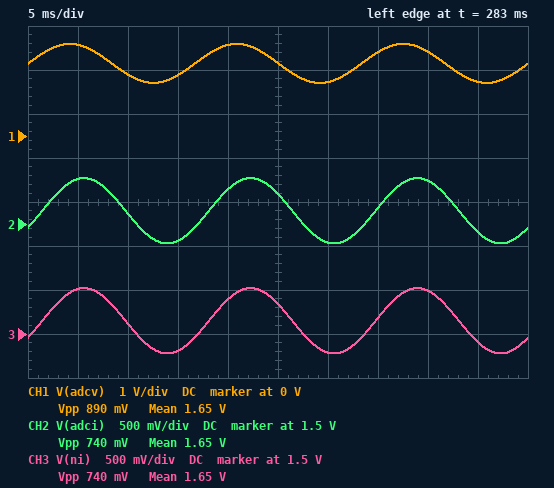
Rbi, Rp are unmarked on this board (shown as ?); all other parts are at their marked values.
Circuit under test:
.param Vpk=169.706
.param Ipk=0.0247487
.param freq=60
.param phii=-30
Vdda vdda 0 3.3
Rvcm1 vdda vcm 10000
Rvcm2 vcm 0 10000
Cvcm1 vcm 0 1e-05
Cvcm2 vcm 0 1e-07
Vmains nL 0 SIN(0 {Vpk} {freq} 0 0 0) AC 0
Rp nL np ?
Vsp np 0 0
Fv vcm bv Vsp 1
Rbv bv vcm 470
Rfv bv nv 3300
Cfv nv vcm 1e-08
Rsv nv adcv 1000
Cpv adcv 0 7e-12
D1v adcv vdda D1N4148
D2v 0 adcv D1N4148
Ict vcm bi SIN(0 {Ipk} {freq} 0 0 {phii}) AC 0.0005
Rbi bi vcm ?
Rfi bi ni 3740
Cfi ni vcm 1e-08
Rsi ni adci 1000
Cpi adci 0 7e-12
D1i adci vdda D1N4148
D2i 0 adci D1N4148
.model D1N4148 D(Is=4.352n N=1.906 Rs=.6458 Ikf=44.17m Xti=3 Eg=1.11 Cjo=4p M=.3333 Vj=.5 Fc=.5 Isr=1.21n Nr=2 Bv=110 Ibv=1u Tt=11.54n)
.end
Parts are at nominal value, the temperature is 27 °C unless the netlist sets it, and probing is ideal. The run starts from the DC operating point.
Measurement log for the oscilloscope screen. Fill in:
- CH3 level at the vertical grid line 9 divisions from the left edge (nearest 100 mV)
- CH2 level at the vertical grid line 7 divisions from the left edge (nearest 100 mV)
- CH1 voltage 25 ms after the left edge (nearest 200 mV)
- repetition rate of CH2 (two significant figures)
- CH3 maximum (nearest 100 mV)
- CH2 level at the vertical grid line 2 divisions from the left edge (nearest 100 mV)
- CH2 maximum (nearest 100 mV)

1.4 V
1.7 V
1.6 V
60 Hz
2.0 V
1.6 V
2.0 V
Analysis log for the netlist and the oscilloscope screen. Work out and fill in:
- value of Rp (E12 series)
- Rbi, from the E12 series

180 kΩ
15 Ω
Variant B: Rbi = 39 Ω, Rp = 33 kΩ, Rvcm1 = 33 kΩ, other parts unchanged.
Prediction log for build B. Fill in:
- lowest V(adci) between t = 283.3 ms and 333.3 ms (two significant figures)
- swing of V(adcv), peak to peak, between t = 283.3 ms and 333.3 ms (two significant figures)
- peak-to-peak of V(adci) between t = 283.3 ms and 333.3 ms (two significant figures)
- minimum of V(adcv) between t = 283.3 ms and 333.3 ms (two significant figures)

85 mV
4.0 V
1.9 V
-520 mV
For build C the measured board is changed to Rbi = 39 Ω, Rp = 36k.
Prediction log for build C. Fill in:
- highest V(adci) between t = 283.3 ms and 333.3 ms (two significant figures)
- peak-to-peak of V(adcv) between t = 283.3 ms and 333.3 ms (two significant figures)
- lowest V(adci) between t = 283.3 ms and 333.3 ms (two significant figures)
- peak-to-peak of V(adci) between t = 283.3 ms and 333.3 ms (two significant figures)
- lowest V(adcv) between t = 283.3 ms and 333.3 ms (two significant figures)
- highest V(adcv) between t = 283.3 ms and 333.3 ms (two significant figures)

2.6 V
4.2 V
690 mV
1.9 V
-430 mV
3.7 V
